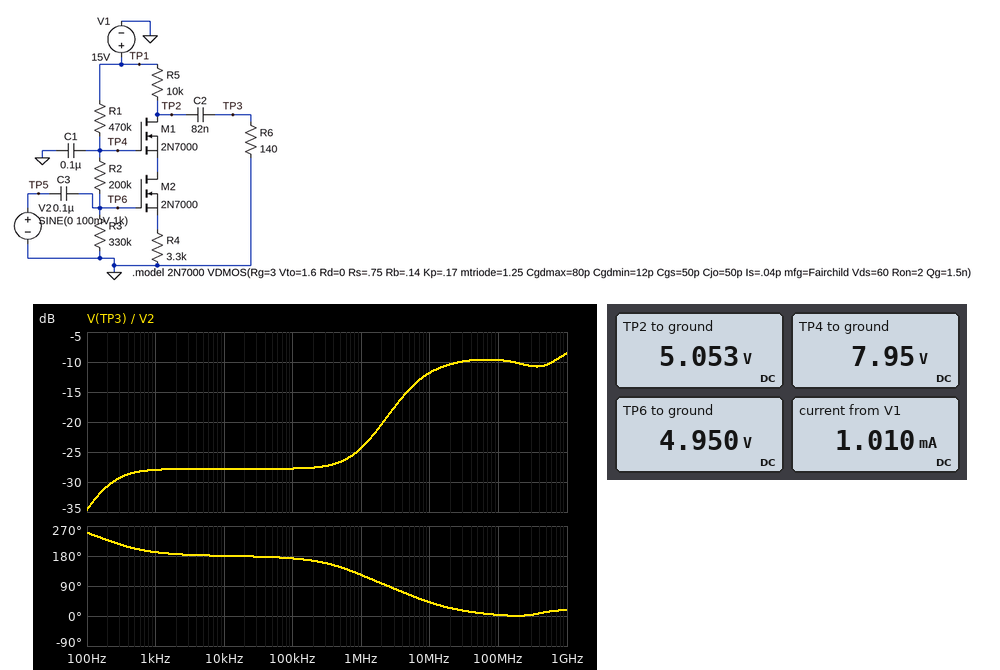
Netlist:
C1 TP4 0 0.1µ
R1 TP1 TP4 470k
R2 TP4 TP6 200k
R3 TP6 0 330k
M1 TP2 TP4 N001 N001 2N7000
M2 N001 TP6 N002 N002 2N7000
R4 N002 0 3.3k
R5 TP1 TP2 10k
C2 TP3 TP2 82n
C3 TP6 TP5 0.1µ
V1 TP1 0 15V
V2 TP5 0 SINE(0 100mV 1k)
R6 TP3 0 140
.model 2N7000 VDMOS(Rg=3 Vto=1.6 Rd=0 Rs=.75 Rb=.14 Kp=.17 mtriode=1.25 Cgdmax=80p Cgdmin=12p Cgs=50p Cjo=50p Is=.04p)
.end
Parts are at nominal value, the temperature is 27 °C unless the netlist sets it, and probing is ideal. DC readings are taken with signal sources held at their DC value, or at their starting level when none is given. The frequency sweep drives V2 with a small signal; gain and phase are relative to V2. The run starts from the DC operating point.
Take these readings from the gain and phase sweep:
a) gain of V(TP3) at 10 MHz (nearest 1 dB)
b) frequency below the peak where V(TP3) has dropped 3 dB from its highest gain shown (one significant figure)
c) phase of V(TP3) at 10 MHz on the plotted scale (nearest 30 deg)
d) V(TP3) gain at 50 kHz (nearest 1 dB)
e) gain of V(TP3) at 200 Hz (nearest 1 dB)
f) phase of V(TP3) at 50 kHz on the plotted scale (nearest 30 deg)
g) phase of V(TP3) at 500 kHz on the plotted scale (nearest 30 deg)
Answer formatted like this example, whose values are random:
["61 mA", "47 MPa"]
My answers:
["-12 dB", "10 MHz", "30 deg", "-28 dB", "-31 dB", "180 deg", "150 deg"]
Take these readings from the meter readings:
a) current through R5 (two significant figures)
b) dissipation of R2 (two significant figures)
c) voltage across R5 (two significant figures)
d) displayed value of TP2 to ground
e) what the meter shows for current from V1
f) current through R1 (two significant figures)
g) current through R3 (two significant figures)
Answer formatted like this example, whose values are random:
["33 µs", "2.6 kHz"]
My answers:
["990 µA", "45 µW", "9.9 V", "5.053 V", "1.010 mA", "15 µA", "15 µA"]
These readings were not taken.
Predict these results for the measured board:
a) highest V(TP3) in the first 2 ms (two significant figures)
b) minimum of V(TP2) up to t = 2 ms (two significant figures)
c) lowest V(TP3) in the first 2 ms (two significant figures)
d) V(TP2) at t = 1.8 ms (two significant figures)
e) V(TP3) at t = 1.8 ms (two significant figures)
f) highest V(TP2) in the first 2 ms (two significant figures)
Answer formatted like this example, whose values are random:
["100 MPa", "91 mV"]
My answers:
["4.3 mV", "5.0 V", "-3.8 mV", "5.1 V", "3.6 mV", "5.1 V"]
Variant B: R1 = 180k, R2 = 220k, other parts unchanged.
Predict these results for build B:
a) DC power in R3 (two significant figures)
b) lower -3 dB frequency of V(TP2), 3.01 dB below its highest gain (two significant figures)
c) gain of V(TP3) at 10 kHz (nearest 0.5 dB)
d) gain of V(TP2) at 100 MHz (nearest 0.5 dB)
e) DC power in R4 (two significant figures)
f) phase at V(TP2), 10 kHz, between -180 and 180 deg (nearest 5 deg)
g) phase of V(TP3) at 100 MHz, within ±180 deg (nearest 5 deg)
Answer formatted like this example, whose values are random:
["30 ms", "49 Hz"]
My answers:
["140 µW", "4.5 MHz", "-59.5 dB", "-6.5 dB", "4.2 mW", "45 deg", "0 deg"]
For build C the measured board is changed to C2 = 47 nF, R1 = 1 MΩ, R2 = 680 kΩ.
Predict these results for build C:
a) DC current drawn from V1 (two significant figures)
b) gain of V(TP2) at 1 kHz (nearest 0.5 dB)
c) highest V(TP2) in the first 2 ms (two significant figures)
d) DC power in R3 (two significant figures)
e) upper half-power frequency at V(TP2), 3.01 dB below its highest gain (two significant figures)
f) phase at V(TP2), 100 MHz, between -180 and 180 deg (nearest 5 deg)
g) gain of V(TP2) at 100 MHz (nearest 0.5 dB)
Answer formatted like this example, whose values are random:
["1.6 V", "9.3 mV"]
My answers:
["280 µA", "-1.0 dB", "12 V", "18 µW", "350 Hz", "10 deg", "-15.5 dB"]
